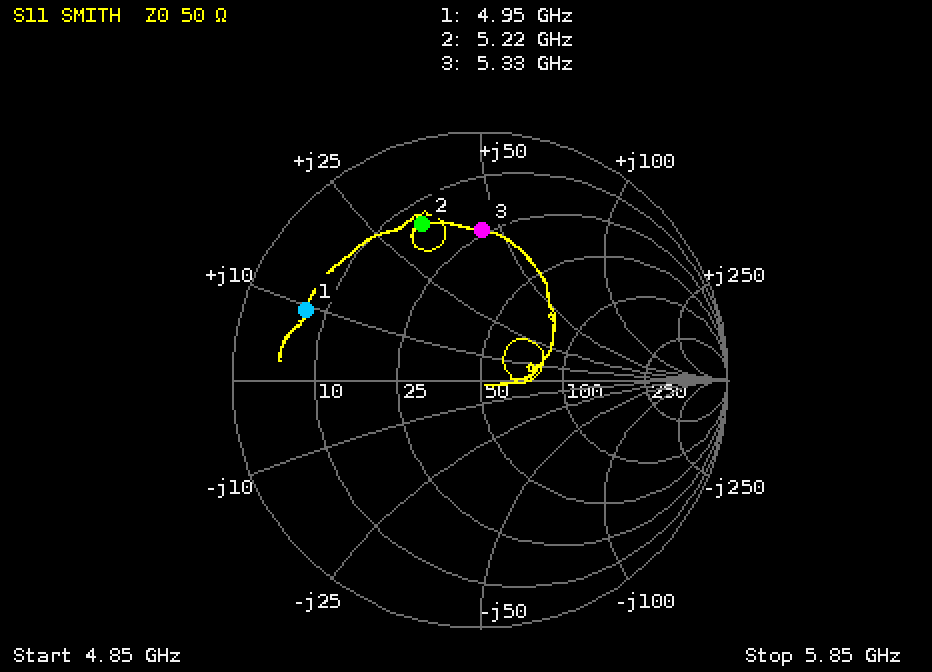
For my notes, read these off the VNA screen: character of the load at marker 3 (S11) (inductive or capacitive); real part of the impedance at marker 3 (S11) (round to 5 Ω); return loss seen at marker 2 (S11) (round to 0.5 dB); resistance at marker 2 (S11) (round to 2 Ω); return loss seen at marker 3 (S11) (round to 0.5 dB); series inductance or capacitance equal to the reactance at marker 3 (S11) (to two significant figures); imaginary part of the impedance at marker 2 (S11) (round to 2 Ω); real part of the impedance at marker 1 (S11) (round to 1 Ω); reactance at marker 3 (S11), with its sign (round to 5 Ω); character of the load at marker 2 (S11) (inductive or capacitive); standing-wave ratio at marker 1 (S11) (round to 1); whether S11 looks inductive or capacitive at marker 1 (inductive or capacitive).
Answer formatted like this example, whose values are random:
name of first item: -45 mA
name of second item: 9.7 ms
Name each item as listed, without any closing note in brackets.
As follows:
character of the load at marker 3 (S11): inductive
real part of the impedance at marker 3 (S11): 25 Ω
return loss seen at marker 2 (S11): 3.5 dB
resistance at marker 2 (S11): 14 Ω
return loss seen at marker 3 (S11): 4.5 dB
series inductance or capacitance equal to the reactance at marker 3 (S11): 1.3 nH
imaginary part of the impedance at marker 2 (S11): +32 Ω
real part of the impedance at marker 1 (S11): 7 Ω
reactance at marker 3 (S11), with its sign: +45 Ω
character of the load at marker 2 (S11): inductive
standing-wave ratio at marker 1 (S11): 7
whether S11 looks inductive or capacitive at marker 1: inductive
